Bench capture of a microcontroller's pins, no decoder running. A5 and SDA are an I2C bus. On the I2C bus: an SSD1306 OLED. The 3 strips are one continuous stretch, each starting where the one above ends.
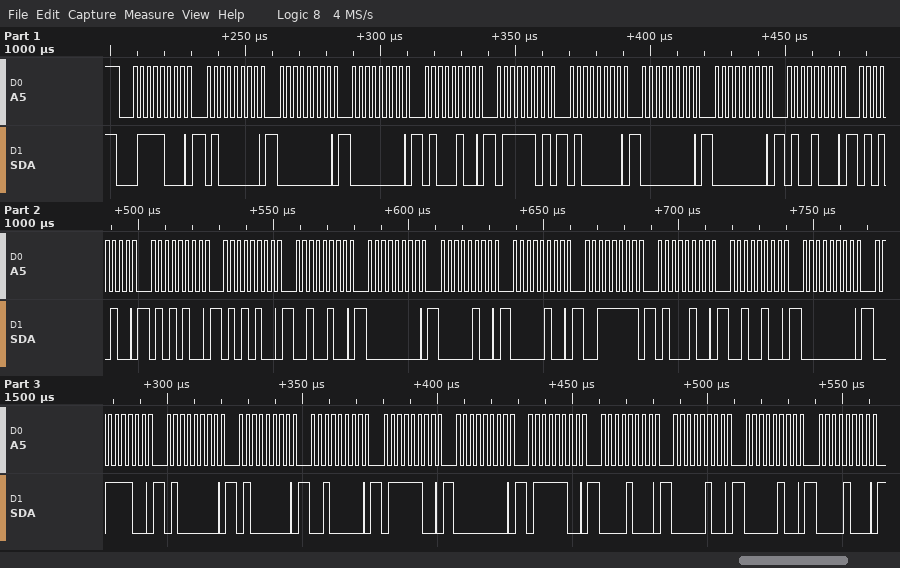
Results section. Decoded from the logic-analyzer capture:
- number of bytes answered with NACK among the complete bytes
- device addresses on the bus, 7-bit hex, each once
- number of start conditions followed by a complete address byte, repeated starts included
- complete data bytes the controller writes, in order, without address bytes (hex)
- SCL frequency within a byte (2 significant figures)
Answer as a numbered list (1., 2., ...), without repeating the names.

1. 0
2. 0x3C
3. 1
4. 40 00 00 44 7D 40 00 00 48 54 54 54 24 00 04 04 3F 44 24 00 3C 40 40 20 7C 00 7C 08 04 04 08
5. 400 kHz
